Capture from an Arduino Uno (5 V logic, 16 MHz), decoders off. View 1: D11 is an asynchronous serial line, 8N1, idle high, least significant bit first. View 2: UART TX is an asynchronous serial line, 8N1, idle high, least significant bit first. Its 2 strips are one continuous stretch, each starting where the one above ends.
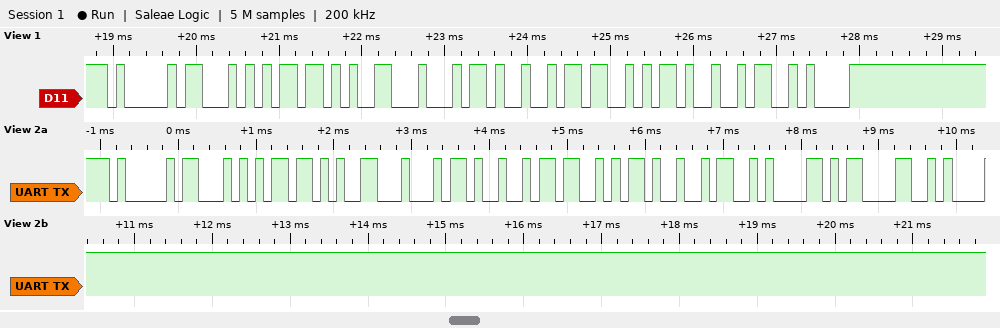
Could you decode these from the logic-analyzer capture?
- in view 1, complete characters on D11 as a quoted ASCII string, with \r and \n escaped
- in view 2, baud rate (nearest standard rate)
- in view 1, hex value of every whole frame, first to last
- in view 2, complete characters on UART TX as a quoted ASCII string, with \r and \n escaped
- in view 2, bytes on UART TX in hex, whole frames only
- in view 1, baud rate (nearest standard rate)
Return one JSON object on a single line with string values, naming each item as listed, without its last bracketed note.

{"in view 1, complete characters on D11 as a quoted ASCII string, with \\r and \\n escaped": "\"AT+DISI\\n\"", "in view 2, baud rate": "9600 baud", "in view 1, hex value of every whole frame, first to last": "0x41 0x54 0x2B 0x44 0x49 0x53 0x49 0x0A", "in view 2, complete characters on UART TX as a quoted ASCII string, with \\r and \\n escaped": "\"AT+DISI\\n\\r\\n\"", "in view 2, bytes on UART TX in hex, whole frames only": "0x41 0x54 0x2B 0x44 0x49 0x53 0x49 0x0A 0x0D 0x0A", "in view 1, baud rate": "9600 baud"}
